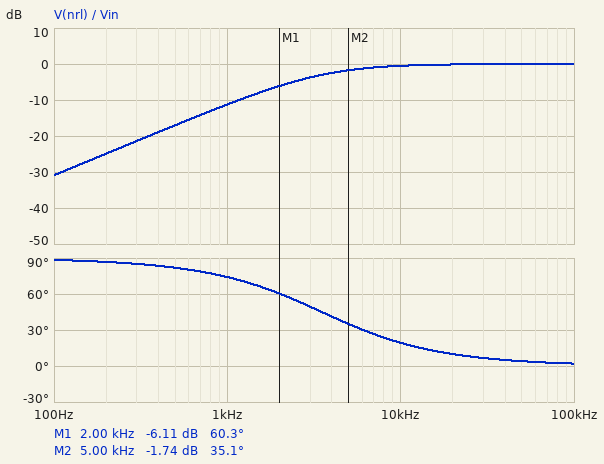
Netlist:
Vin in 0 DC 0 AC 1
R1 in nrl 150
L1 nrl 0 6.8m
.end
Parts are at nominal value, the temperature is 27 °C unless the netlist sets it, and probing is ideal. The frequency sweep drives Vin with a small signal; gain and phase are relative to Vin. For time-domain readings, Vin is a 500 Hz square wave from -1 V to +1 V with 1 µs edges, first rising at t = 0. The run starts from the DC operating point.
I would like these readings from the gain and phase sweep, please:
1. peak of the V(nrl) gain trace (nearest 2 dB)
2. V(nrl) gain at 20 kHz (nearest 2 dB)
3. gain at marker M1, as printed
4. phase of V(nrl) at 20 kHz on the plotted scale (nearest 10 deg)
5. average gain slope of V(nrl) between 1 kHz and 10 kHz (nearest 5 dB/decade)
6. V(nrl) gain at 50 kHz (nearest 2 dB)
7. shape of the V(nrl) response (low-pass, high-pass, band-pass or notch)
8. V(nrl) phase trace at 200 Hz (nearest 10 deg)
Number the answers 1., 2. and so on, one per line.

1. 0 dB
2. 0 dB
3. -6.11 dB
4. 10 deg
5. 10 dB/decade
6. 0 dB
7. high-pass
8. 90 deg
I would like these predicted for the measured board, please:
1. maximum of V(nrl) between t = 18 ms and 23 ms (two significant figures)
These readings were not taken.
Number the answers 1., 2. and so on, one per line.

1. 2.0 V
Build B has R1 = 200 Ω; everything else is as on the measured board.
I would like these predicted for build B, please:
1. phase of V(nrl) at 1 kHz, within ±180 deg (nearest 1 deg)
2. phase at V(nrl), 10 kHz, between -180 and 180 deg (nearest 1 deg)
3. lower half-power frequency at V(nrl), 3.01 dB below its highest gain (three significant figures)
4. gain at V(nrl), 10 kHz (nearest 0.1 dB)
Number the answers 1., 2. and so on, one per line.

1. 78 deg
2. 25 deg
3. 4.68 kHz
4. -0.9 dB
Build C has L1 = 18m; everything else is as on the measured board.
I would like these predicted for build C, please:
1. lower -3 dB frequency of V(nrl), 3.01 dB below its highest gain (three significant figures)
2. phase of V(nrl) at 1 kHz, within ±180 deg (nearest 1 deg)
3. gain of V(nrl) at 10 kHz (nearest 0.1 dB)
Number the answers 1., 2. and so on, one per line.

1. 1.33 kHz
2. 53 deg
3. -0.1 dB
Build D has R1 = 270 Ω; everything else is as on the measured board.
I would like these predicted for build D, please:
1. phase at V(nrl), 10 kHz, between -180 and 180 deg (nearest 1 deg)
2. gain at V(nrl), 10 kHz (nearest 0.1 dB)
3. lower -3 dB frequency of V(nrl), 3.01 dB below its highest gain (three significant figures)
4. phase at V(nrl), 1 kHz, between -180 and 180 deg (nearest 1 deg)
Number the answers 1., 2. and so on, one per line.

1. 32 deg
2. -1.5 dB
3. 6.32 kHz
4. 81 deg
